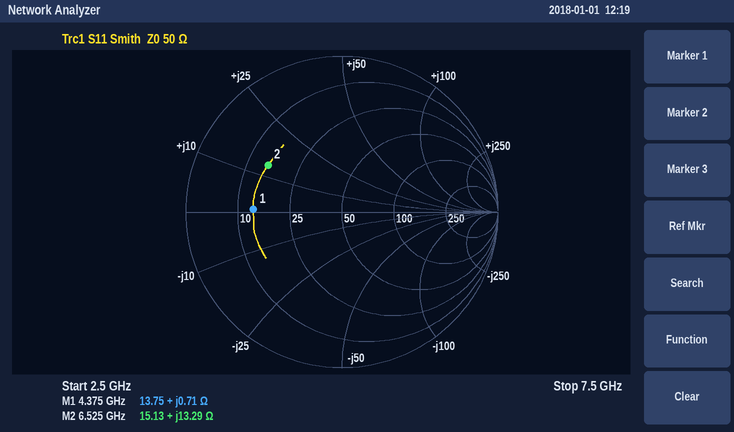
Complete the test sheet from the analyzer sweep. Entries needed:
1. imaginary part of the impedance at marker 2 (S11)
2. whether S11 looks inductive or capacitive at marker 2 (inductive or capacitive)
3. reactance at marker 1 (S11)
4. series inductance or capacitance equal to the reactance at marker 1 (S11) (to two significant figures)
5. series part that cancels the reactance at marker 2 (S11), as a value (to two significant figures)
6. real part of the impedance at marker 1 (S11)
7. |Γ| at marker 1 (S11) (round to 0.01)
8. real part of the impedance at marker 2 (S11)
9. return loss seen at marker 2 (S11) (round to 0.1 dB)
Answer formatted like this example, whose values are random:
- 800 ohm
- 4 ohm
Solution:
- +13.29 Ω
- inductive
- +0.71 Ω
- 26 pH
- 1.8 pF
- 13.75 Ω
- 0.57
- 15.13 Ω
- 5.0 dB
